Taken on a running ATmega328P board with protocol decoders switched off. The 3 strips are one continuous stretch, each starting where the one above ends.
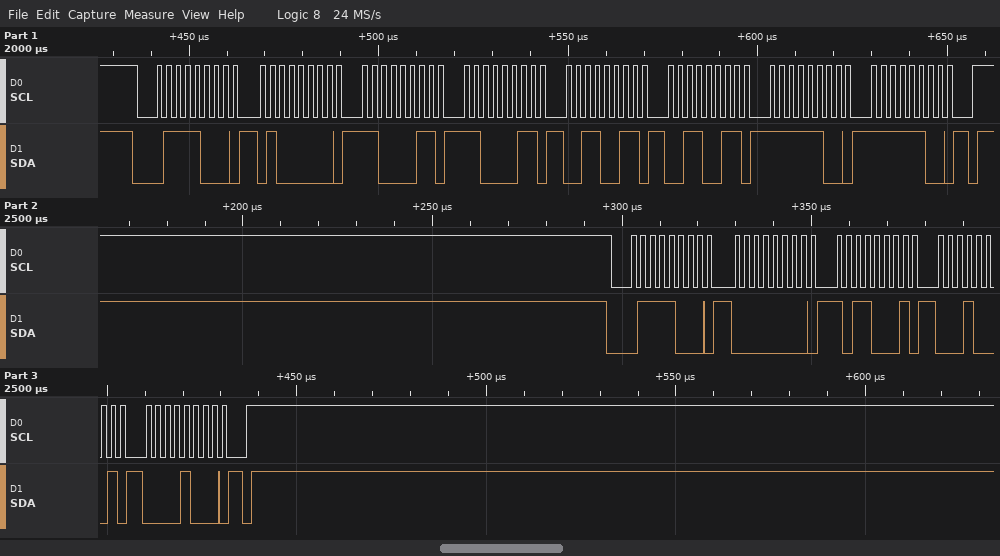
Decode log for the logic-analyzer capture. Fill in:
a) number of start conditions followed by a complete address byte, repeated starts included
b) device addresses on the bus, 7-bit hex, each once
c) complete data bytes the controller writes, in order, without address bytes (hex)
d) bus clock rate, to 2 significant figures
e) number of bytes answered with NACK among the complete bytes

2
0x3C
40 C3 C3 33 33 FC FC 00 B1 11 08
400 kHz
0
